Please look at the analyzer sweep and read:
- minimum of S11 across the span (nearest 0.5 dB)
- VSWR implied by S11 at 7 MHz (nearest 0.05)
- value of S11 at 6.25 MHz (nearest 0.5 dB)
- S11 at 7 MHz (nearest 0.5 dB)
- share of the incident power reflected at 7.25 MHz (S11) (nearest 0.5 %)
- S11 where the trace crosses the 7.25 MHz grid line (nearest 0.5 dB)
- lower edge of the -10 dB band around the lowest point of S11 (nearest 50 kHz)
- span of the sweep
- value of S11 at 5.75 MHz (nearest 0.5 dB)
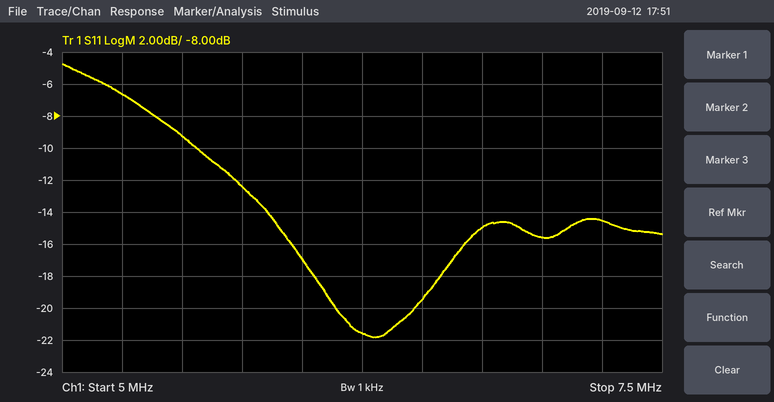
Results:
-22.0 dB
1.40
-21.5 dB
-15.5 dB
3.5 %
-14.5 dB
5.55 MHz
2.5 MHz
-12.5 dB
